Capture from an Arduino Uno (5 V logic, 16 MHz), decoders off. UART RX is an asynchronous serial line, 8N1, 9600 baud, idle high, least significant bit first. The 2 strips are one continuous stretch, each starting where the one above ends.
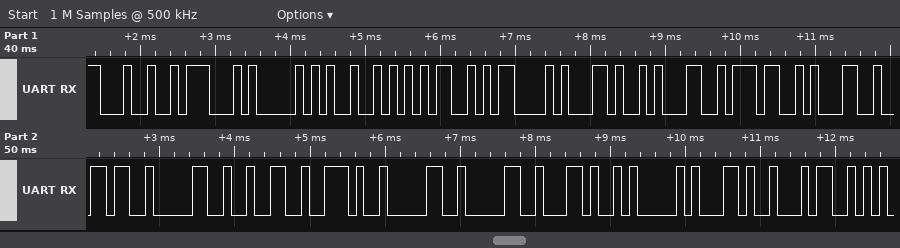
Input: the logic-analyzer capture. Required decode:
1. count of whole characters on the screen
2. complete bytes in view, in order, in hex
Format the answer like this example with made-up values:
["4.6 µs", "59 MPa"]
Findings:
["20", "0x24 0x47 0x50 0x52 0x4D 0x43 0x2C 0x31 0x37 0x31 0x36 0x30 0x32 0x2E 0x30 0x30 0x2C 0x41 0x2C 0x34"]
